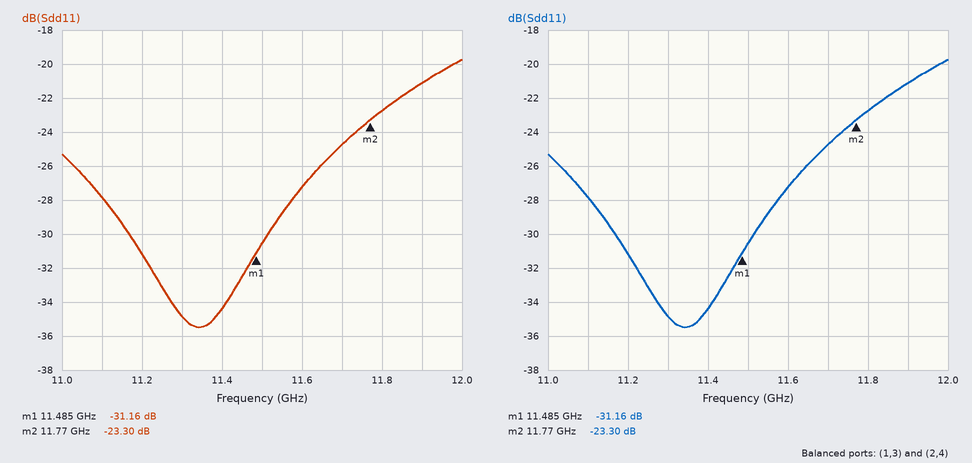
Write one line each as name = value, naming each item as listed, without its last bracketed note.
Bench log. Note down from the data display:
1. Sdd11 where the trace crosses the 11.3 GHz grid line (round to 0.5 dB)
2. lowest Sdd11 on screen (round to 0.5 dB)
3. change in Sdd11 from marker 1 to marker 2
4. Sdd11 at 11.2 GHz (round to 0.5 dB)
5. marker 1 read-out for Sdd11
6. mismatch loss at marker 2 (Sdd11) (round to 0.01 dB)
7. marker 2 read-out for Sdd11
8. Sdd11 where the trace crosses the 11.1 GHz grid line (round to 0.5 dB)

Sdd11 where the trace crosses the 11.3 GHz grid line = -35.0 dB
lowest Sdd11 on screen = -35.5 dB
change in Sdd11 from marker 1 to marker 2 = 7.86 dB
Sdd11 at 11.2 GHz = -31.0 dB
marker 1 read-out for Sdd11 = -31.16 dB
mismatch loss at marker 2 (Sdd11) = 0.02 dB
marker 2 read-out for Sdd11 = -23.30 dB
Sdd11 where the trace crosses the 11.1 GHz grid line = -28.0 dB
